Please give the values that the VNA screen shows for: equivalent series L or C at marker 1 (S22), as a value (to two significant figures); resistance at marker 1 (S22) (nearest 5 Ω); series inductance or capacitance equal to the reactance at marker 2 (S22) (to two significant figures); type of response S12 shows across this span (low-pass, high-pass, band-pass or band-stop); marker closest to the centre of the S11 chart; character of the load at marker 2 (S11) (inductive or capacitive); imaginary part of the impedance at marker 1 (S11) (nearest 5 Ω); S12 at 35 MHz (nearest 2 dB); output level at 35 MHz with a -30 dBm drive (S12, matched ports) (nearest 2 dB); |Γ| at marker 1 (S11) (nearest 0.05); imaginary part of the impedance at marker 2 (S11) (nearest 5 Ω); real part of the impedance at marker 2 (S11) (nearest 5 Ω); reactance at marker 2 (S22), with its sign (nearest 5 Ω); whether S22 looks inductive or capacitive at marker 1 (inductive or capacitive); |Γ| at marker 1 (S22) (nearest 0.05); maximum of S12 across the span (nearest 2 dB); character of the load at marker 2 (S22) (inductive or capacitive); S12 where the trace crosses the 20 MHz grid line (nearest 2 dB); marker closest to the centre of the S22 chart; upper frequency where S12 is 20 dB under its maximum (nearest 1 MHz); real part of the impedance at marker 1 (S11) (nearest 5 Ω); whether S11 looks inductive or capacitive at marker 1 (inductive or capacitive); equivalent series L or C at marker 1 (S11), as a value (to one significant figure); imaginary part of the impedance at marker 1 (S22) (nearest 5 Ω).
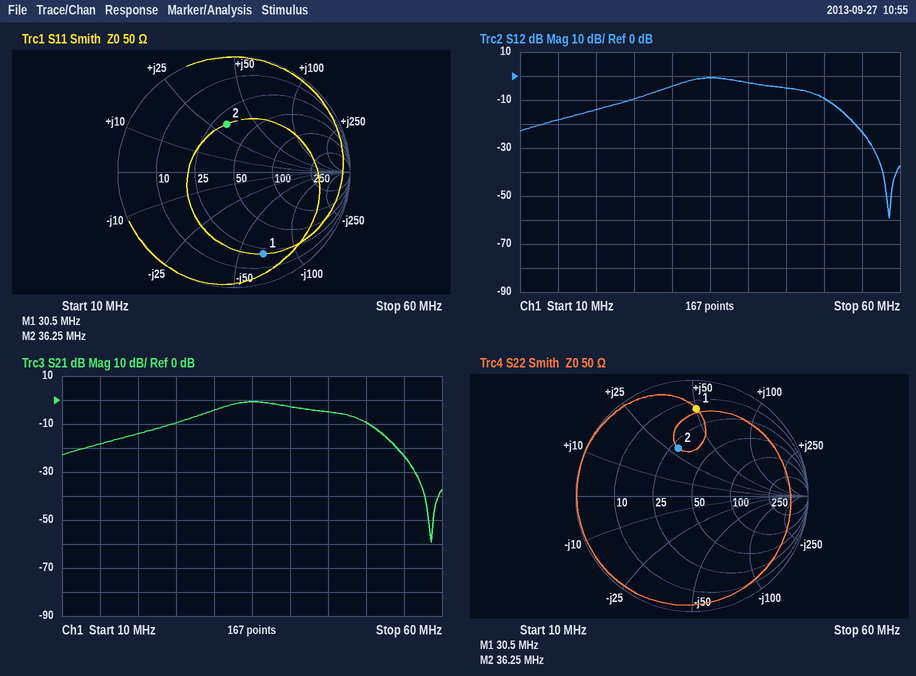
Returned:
260 nH
15 Ω
130 nH
band-pass
marker 2
inductive
-65 Ω
0 dB
-30 dBm
0.75
+30 Ω
30 Ω
+30 Ω
inductive
0.75
0 dB
inductive
-14 dB
marker 2
54 MHz
20 Ω
capacitive
80 pF
+50 Ω
